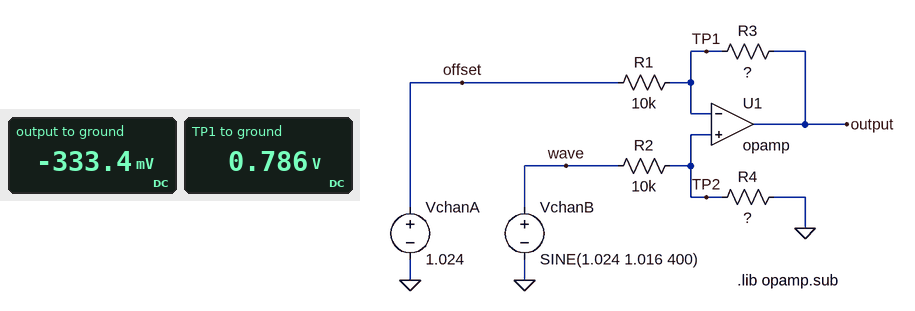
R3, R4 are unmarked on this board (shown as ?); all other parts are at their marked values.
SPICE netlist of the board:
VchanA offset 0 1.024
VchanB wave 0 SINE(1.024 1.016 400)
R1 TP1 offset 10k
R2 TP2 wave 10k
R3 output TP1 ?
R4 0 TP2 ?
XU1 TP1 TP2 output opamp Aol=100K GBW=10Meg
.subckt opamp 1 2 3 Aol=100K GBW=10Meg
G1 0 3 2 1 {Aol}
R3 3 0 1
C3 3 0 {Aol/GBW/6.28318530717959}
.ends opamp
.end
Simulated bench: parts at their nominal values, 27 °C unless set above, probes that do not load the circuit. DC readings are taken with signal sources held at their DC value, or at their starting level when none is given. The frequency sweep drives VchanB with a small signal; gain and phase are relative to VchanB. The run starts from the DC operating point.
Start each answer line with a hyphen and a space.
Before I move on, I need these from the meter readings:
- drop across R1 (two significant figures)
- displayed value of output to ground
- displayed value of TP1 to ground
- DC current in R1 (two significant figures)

- 240 mV
- -333.4 mV
- 0.786 V
- 24 µA
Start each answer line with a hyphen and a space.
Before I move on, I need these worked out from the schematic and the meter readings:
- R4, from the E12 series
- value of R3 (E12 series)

- 33 kΩ
- 47 kΩ
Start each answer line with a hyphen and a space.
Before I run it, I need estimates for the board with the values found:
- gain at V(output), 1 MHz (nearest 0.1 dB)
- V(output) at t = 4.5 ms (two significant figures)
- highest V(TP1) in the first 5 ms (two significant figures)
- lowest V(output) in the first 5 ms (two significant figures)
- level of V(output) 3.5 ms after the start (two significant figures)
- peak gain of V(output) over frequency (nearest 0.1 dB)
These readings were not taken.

- 11.6 dB
- -4.6 V
- 1.6 V
- -4.8 V
- 2.3 V
- 12.8 dB
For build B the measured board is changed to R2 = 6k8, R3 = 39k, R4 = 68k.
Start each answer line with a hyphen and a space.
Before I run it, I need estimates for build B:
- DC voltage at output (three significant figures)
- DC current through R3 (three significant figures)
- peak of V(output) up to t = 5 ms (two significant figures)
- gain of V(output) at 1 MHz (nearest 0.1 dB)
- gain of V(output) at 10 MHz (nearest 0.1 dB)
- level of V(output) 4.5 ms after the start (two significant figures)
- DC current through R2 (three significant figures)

- 568 mV
- 9.31 µA
- 5.1 V
- 12.0 dB
- -1.0 dB
- -3.7 V
- 13.7 µA
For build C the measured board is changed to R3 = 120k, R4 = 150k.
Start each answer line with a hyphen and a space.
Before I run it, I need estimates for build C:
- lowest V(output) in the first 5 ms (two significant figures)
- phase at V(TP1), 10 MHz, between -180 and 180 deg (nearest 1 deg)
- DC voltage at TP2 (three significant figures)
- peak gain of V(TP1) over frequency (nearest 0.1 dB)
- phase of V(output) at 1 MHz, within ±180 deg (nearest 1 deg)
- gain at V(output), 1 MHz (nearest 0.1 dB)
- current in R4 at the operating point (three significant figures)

- -12 V
- -86 deg
- 960 mV
- -0.6 dB
- -52 deg
- 17.4 dB
- 6.40 µA
